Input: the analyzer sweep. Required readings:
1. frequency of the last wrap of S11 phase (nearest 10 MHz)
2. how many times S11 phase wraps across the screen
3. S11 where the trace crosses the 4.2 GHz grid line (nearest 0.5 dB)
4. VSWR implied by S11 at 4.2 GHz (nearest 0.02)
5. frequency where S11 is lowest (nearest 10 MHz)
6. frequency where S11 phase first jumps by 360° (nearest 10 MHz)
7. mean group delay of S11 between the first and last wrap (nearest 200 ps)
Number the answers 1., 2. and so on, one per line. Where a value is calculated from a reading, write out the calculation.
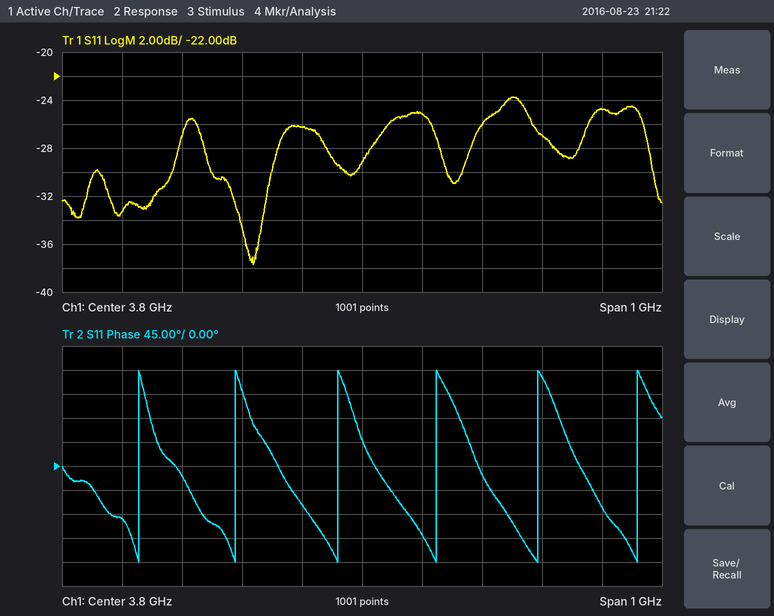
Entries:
1. 4.26 GHz
2. 6
3. -25.0 dB
4. |Γ| = 10^(-25/20) = 0.0562; VSWR = (1 + 0.0562)/(1 − 0.0562) ≈ 1.12
5. 3.62 GHz
6. 3.43 GHz
7. 5 cycles / (4.26 GHz − 3.43 GHz) ≈ 6.0 ns
